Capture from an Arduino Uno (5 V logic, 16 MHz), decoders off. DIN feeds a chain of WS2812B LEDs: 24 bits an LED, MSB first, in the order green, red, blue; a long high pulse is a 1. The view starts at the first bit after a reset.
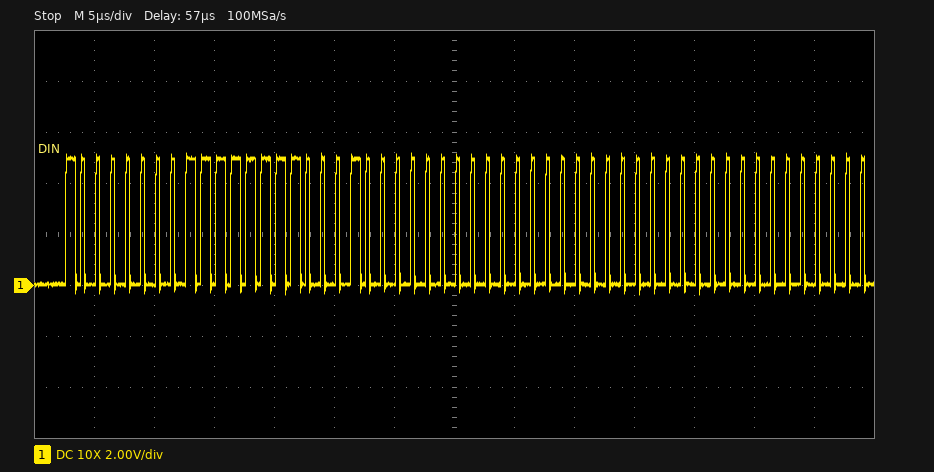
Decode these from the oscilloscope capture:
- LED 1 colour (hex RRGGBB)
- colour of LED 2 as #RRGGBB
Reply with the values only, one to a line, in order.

#FF8010
#000000
